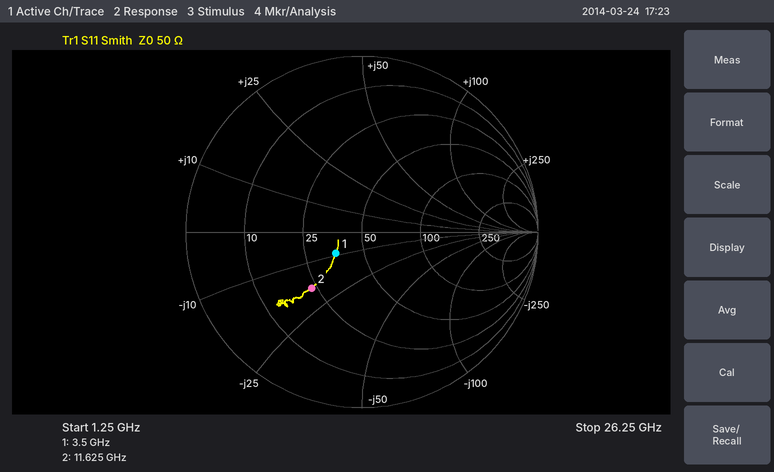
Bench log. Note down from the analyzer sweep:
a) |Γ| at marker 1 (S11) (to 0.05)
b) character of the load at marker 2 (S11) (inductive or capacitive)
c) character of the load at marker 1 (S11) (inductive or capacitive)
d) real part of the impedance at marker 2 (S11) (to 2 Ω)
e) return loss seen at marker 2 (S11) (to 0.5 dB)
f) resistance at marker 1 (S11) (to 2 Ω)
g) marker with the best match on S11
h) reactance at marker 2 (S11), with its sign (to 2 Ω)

0.20
capacitive
capacitive
24 Ω
7.5 dB
36 Ω
marker 1
-18 Ω
